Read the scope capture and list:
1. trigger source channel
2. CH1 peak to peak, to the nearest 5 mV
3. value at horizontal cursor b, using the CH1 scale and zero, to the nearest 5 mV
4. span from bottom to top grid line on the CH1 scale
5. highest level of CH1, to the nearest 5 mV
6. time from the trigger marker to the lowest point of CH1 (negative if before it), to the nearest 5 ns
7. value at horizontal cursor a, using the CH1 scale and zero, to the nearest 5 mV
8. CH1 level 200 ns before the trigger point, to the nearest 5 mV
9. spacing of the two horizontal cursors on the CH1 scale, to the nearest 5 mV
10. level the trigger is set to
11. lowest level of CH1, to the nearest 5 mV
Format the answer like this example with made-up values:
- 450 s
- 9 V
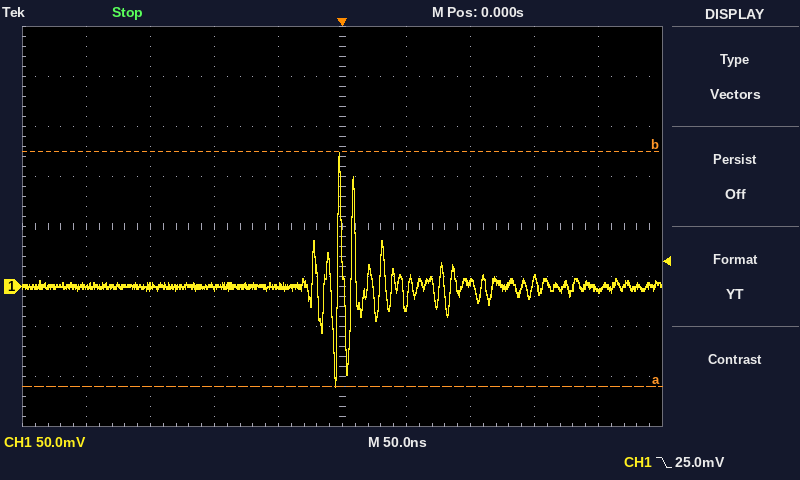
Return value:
- CH1
- 235 mV
- 135 mV
- 400 mV
- 135 mV
- -5 ns
- -100 mV
- 0 mV
- 235 mV
- 25.0 mV
- -100 mV
